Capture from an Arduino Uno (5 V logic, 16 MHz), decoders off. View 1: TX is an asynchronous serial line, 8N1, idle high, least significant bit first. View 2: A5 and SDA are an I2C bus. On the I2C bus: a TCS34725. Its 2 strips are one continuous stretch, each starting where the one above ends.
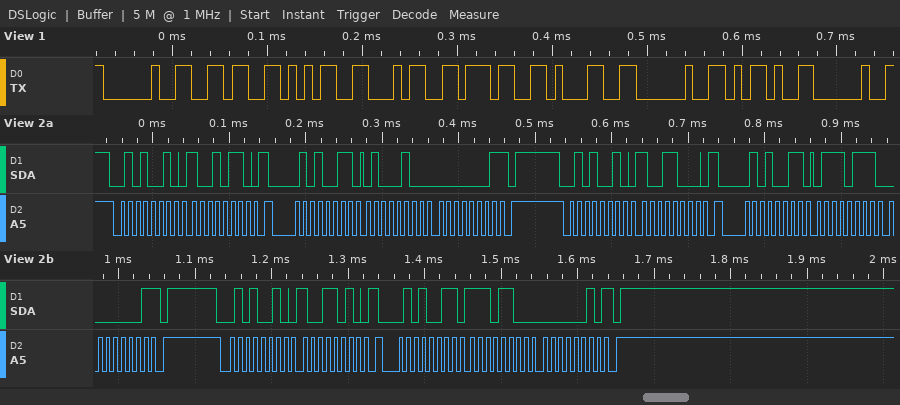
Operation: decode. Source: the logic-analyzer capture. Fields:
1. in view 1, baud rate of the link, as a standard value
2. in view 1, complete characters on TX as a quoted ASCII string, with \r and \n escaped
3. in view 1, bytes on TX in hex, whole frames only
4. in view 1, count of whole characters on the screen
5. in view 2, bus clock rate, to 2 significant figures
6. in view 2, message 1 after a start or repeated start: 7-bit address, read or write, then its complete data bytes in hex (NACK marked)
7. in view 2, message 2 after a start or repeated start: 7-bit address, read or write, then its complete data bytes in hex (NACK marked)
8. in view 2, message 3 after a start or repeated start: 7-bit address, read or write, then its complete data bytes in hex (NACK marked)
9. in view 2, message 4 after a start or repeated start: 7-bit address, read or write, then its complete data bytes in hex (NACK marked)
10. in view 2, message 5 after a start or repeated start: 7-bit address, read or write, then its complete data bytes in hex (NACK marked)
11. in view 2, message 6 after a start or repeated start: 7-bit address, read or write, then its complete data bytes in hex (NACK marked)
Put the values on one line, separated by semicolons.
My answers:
115200 baud; " 65471 - "; 20 36 35 34 37 31 20 2D 20; 9; 100 kHz; 0x29 write: 96; 0x29 read: 44 01 NACK; 0x29 write: 98; 0x29 read: 77 01 NACK; 0x29 write: 9A; 0x29 read: EC 02 NACK
